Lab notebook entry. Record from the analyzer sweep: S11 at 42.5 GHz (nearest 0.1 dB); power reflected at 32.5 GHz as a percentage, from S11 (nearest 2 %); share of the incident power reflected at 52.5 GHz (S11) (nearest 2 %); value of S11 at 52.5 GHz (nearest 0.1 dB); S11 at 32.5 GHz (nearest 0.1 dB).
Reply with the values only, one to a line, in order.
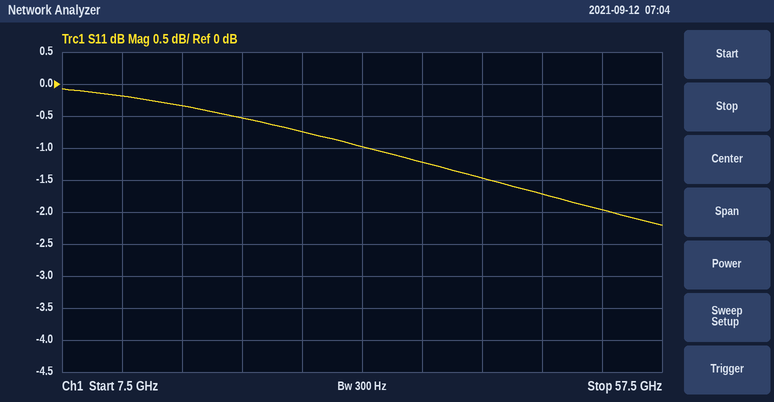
-1.5 dB
80 %
64 %
-2.0 dB
-1.0 dB
